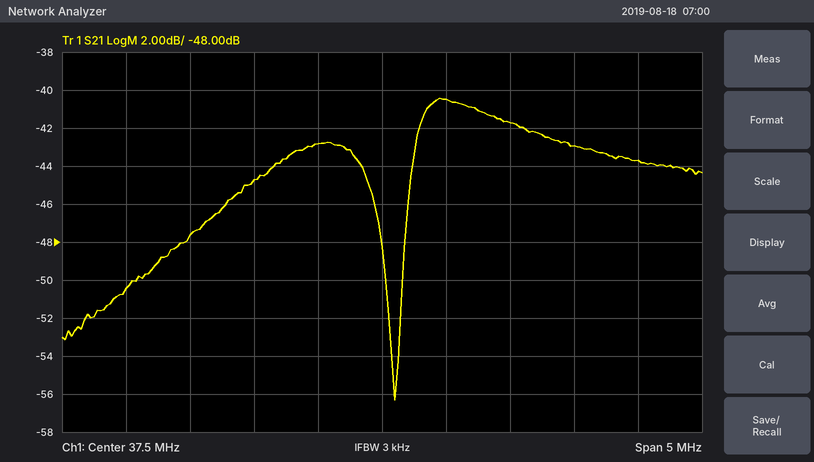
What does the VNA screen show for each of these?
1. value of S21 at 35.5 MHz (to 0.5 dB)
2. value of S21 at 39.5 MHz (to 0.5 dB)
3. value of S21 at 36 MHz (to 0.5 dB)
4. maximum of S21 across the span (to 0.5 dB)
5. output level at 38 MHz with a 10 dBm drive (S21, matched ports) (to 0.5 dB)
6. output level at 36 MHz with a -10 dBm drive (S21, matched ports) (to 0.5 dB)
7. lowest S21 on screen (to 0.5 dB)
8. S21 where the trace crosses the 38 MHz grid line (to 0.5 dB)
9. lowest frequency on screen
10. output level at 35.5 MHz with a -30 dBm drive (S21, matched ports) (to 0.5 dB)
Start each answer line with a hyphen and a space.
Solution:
- -50.5 dB
- -43.5 dB
- -47.5 dB
- -40.5 dB
- -30.5 dBm
- -57.5 dBm
- -56.5 dB
- -40.5 dB
- 35 MHz
- -80.5 dBm
